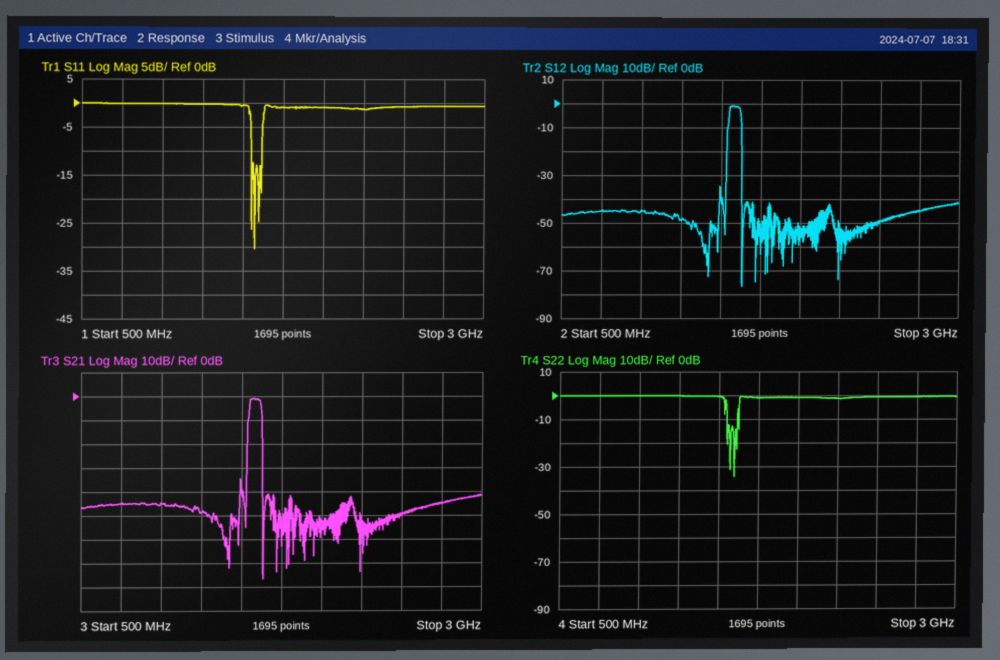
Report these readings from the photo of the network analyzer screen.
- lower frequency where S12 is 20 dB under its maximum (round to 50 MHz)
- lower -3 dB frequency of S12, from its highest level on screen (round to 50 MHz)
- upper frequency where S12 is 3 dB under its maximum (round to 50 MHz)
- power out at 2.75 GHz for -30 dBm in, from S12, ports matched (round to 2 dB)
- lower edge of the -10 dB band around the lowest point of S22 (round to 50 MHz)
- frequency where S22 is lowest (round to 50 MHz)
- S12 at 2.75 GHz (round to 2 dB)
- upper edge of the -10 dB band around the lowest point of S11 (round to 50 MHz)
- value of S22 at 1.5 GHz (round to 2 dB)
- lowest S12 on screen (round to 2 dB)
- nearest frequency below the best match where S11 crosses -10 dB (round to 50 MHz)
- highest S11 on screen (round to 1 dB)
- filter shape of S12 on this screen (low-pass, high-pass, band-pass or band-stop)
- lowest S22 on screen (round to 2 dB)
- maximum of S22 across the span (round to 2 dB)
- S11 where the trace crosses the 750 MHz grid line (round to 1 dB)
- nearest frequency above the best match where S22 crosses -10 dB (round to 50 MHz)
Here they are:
1.55 GHz
1.55 GHz
1.60 GHz
-74 dBm
1.55 GHz
1.60 GHz
-44 dB
1.60 GHz
0 dB
-76 dB
1.55 GHz
0 dB
band-pass
-34 dB
0 dB
0 dB
1.60 GHz
